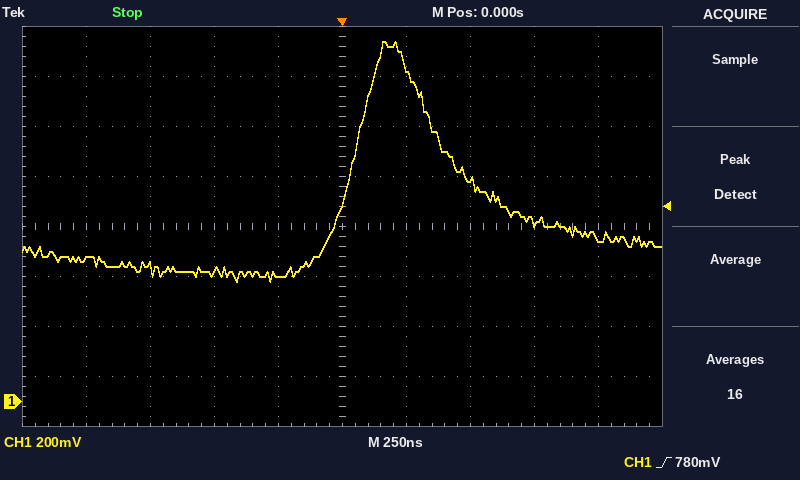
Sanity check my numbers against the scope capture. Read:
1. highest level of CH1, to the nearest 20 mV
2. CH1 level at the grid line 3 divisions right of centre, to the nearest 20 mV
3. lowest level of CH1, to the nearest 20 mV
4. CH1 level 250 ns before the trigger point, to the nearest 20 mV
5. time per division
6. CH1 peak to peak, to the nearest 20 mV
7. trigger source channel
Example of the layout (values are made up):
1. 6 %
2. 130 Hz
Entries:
1. 1.44 V
2. 720 mV
3. 480 mV
4. 500 mV
5. 250 ns
6. 960 mV
7. CH1
